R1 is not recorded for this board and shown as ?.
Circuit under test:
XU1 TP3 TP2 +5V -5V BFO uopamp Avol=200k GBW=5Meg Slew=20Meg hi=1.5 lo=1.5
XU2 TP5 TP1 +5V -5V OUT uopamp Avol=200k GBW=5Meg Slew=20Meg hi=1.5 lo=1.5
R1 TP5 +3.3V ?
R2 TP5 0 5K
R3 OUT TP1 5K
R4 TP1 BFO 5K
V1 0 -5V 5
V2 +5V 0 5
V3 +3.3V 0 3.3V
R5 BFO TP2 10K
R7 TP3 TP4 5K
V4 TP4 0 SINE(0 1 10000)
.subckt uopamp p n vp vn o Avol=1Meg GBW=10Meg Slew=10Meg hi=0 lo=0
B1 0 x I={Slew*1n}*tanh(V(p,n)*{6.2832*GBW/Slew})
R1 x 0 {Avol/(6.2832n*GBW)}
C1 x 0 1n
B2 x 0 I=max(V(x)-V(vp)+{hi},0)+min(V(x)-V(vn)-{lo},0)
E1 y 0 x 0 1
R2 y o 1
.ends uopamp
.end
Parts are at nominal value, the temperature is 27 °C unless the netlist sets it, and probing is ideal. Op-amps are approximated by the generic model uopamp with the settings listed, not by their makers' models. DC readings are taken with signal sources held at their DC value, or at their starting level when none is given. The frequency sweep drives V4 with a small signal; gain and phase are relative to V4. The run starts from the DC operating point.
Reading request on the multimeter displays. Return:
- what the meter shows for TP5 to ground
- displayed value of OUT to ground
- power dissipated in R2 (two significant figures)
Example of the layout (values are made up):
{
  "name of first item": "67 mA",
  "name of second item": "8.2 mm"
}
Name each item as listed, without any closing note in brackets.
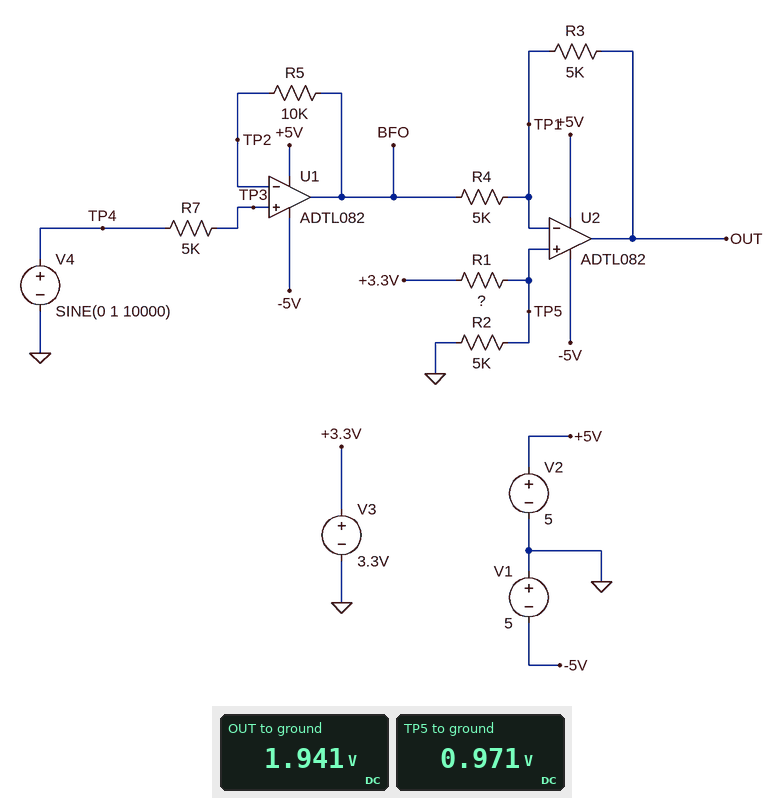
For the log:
{
  "what the meter shows for TP5 to ground": "0.971 V",
  "displayed value of OUT to ground": "1.941 V",
  "power dissipated in R2": "190 µW"
}
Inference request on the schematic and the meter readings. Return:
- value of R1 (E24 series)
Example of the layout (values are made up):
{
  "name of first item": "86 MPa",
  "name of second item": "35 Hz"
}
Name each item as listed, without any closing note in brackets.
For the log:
{
  "value of R1": "12 kΩ"
}
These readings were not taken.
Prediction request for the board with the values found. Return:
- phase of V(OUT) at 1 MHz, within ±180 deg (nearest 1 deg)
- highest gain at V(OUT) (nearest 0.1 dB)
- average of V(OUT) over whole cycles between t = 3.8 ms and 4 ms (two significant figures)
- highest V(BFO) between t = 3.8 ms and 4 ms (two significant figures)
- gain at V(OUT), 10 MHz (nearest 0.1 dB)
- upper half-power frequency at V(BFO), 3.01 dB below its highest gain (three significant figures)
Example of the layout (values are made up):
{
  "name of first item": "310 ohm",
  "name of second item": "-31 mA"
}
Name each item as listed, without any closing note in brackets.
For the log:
{
  "phase of V(OUT) at 1 MHz, within ±180 deg": "147 deg",
  "highest gain at V(OUT)": "0 dB",
  "average of V(OUT) over whole cycles between t = 3.8 ms and 4 ms": "1.9 V",
  "highest V(BFO) between t = 3.8 ms and 4 ms": "1.0 V",
  "gain at V(OUT), 10 MHz": "-19.3 dB",
  "upper half-power frequency at V(BFO), 3.01 dB below its highest gain": "5.00 MHz"
}
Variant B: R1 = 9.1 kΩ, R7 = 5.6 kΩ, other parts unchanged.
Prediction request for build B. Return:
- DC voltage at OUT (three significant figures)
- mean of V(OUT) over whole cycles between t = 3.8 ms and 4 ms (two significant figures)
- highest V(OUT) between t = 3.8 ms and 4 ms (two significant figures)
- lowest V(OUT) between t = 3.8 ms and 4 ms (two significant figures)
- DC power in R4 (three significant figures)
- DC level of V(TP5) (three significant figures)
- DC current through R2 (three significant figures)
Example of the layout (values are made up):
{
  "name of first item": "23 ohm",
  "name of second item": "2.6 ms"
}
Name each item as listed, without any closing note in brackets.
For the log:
{
  "DC voltage at OUT": "2.34 V",
  "mean of V(OUT) over whole cycles between t = 3.8 ms and 4 ms": "2.3 V",
  "highest V(OUT) between t = 3.8 ms and 4 ms": "3.3 V",
  "lowest V(OUT) between t = 3.8 ms and 4 ms": "1.3 V",
  "DC power in R4": "274 µW",
  "DC level of V(TP5)": "1.17 V",
  "DC current through R2": "234 µA"
}
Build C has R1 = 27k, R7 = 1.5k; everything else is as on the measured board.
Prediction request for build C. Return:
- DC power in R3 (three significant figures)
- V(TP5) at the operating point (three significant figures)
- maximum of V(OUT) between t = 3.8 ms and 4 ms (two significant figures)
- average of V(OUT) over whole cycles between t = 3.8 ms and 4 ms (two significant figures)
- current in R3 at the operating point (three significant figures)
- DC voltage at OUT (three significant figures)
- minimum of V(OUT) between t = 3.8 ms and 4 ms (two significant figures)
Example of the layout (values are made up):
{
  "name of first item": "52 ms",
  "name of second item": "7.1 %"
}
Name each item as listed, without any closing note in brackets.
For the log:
{
  "DC power in R3": "53.2 µW",
  "V(TP5) at the operating point": "516 mV",
  "maximum of V(OUT) between t = 3.8 ms and 4 ms": "2.0 V",
  "average of V(OUT) over whole cycles between t = 3.8 ms and 4 ms": "1.0 V",
  "current in R3 at the operating point": "103 µA",
  "DC voltage at OUT": "1.03 V",
  "minimum of V(OUT) between t = 3.8 ms and 4 ms": "31 mV"
}
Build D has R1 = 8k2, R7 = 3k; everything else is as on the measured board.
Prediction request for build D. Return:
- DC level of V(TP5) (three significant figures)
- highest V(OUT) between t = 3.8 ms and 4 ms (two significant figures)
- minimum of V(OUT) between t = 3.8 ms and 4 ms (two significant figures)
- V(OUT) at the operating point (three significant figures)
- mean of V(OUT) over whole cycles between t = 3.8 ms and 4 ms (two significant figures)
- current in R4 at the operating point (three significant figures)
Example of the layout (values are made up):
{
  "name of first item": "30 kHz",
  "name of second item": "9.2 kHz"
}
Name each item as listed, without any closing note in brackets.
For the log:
{
  "DC level of V(TP5)": "1.25 V",
  "highest V(OUT) between t = 3.8 ms and 4 ms": "3.5 V",
  "minimum of V(OUT) between t = 3.8 ms and 4 ms": "1.5 V",
  "V(OUT) at the operating point": "2.50 V",
  "mean of V(OUT) over whole cycles between t = 3.8 ms and 4 ms": "2.5 V",
  "current in R4 at the operating point": "250 µA"
}
